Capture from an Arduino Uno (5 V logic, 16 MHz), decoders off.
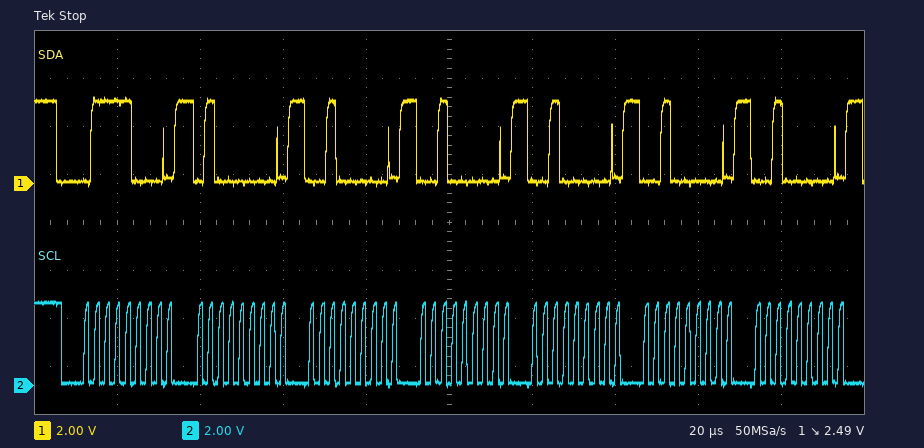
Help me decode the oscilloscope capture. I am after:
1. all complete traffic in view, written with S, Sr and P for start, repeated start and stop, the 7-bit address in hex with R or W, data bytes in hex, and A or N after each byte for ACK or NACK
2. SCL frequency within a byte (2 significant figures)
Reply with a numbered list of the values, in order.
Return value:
1. S 3CW A 40 A 20 A 20 A 20 A 20 A 20 A
2. 400 kHz
